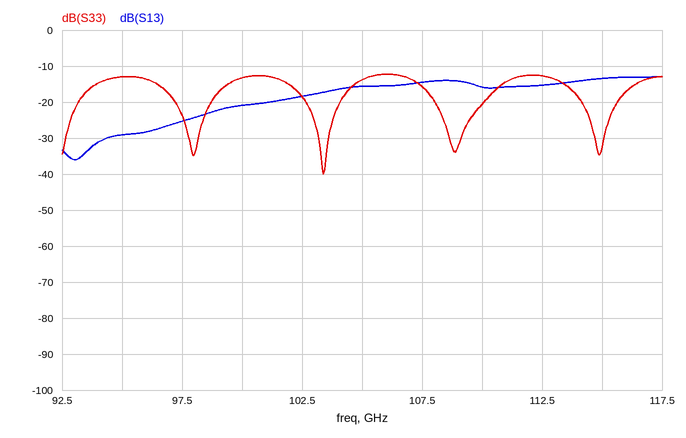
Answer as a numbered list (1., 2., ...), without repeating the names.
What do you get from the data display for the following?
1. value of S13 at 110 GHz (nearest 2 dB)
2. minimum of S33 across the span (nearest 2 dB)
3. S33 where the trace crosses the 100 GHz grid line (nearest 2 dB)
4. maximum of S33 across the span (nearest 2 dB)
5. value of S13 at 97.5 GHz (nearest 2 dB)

1. -16 dB
2. -40 dB
3. -14 dB
4. -12 dB
5. -26 dB
